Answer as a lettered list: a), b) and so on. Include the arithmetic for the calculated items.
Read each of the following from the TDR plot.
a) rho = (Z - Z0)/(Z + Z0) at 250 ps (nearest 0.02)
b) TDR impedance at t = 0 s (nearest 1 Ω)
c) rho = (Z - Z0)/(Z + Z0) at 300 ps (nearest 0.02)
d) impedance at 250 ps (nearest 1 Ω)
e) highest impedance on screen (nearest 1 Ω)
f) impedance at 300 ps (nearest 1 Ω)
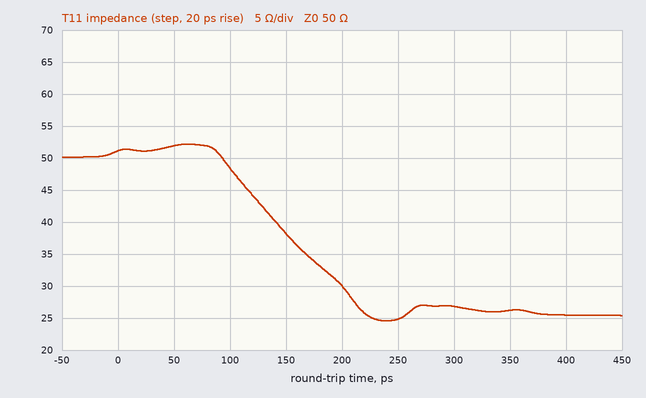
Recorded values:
a) (25 − 50)/(25 + 50) ≈ -0.333, so -0.34 to the nearest 0.02
b) 51 Ω
c) (27 − 50)/(27 + 50) ≈ -0.30
d) 25 Ω
e) 52 Ω
f) 27 Ω
